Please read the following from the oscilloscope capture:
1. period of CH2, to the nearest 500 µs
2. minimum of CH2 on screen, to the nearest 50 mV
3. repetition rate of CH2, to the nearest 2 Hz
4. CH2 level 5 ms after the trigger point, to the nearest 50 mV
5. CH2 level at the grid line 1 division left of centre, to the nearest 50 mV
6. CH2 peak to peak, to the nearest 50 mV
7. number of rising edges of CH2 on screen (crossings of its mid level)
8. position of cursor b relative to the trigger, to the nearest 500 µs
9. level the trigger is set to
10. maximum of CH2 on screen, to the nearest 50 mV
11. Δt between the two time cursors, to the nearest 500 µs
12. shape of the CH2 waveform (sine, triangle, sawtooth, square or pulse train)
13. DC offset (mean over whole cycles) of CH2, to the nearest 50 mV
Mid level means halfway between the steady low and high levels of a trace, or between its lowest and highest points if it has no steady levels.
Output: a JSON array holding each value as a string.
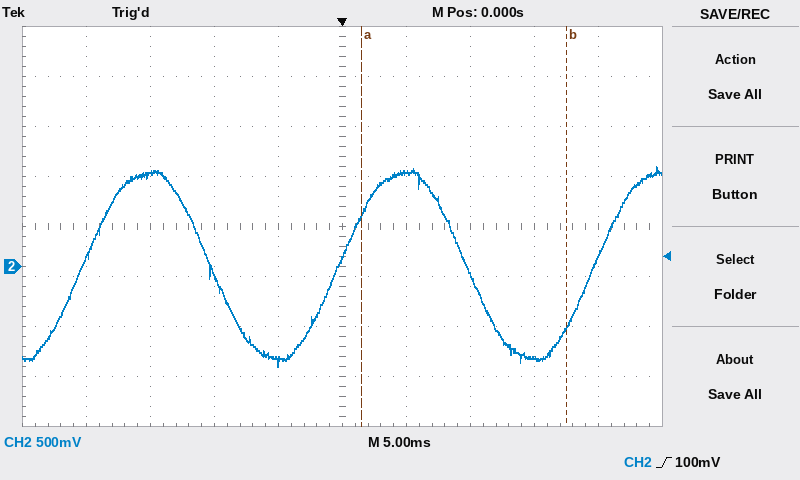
["20.0 ms", "-1.00 V", "50 Hz", "950 mV", "-950 mV", "2.00 V", "3", "+17.5 ms", "100 mV", "1.00 V", "16.0 ms", "sine", "0 mV"]
